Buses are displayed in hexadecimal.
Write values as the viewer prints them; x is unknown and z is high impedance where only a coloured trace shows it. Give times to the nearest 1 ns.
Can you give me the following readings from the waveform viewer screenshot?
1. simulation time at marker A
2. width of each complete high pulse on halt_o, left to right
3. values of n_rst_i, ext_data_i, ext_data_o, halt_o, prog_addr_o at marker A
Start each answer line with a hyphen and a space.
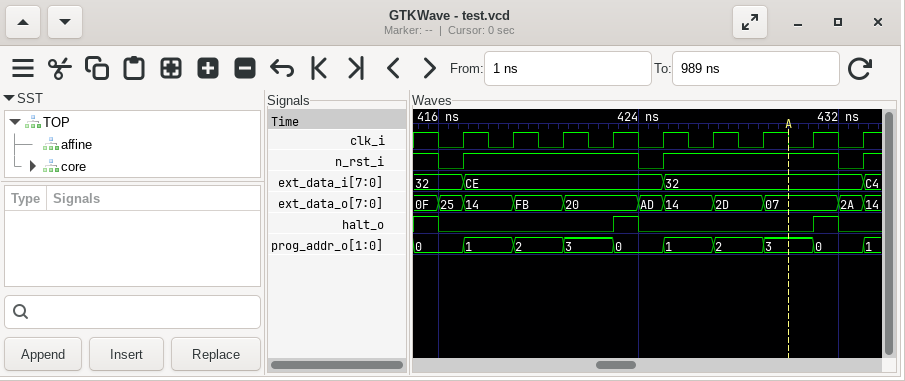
- 430 ns
- 1 ns, 1 ns
- n_rst_i=1, ext_data_i=32, ext_data_o=07, halt_o=0, prog_addr_o=3
